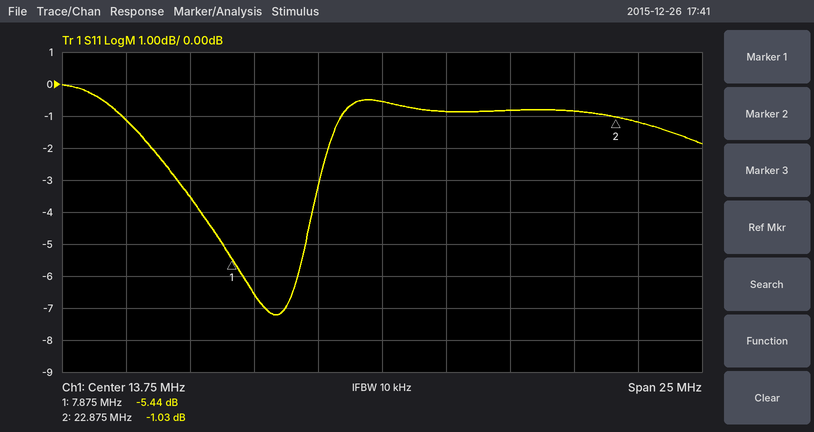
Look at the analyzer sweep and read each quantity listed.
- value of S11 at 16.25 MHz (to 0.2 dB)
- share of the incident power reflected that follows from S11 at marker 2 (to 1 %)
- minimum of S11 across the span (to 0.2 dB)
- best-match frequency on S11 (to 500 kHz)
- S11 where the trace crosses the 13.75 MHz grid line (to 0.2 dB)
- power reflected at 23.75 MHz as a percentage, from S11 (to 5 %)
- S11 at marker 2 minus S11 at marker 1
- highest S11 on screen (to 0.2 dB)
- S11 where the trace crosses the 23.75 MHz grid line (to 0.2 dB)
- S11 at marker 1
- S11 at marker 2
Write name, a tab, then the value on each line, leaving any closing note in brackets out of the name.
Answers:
value of S11 at 16.25 MHz	-0.8 dB
share of the incident power reflected that follows from S11 at marker 2	79 %
minimum of S11 across the span	-7.2 dB
best-match frequency on S11	9.5 MHz
S11 where the trace crosses the 13.75 MHz grid line	-0.6 dB
power reflected at 23.75 MHz as a percentage, from S11	75 %
S11 at marker 2 minus S11 at marker 1	4.41 dB
highest S11 on screen	0.0 dB
S11 where the trace crosses the 23.75 MHz grid line	-1.2 dB
S11 at marker 1	-5.44 dB
S11 at marker 2	-1.03 dB
